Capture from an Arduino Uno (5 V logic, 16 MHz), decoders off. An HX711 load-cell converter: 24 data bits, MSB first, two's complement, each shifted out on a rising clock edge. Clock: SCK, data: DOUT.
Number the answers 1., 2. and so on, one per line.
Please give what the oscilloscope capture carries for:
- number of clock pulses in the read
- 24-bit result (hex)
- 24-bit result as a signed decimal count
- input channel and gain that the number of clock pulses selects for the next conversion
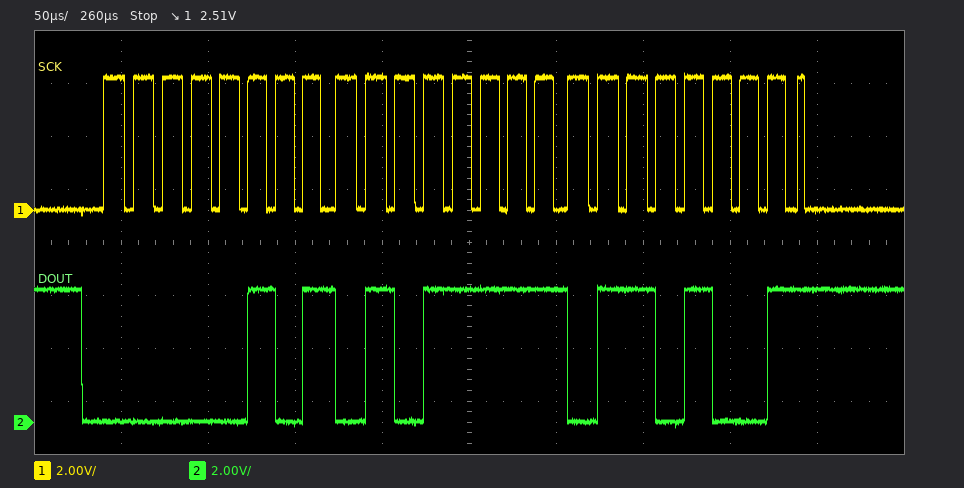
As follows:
1. 25
2. 0x055F69
3. 352105
4. channel A, gain 128
